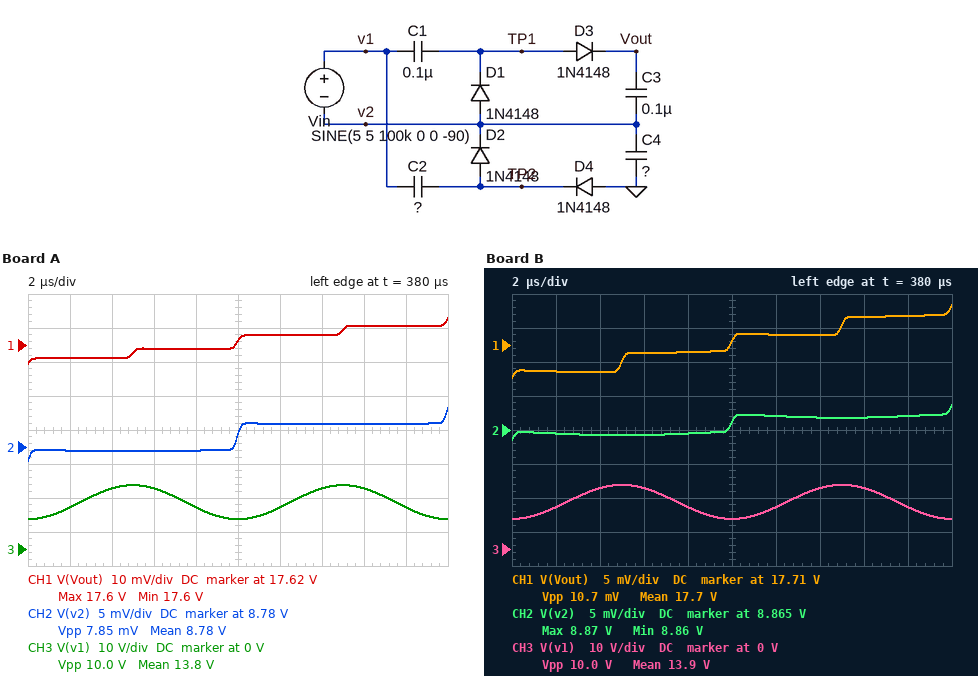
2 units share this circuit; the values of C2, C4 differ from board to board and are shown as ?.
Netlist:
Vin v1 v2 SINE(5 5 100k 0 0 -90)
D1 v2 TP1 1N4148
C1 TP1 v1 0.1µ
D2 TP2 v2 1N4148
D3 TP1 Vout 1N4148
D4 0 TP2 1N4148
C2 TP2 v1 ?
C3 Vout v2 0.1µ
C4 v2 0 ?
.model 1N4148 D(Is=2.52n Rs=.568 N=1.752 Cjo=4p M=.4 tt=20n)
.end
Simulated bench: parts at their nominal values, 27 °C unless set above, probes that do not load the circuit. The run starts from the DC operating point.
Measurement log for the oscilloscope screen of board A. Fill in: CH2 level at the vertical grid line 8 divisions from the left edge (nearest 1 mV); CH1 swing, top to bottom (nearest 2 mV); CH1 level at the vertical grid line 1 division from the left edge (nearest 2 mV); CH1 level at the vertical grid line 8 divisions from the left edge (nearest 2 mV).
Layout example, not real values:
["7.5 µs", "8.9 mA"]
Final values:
["8.783 V", "14 mV", "17.616 V", "17.626 V"]
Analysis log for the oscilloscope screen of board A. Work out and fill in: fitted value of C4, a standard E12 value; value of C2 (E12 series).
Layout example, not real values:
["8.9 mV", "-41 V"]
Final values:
["150 nF", "47 nF"]
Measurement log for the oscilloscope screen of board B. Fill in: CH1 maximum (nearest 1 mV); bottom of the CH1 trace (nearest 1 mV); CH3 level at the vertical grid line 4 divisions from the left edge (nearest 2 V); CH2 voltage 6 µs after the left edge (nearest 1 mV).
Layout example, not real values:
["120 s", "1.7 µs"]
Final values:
["17.711 V", "17.700 V", "12 V", "8.864 V"]
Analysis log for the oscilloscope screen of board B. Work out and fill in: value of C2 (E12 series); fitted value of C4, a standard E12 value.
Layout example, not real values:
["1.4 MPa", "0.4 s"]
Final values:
["330 nF", "47 nF"]
